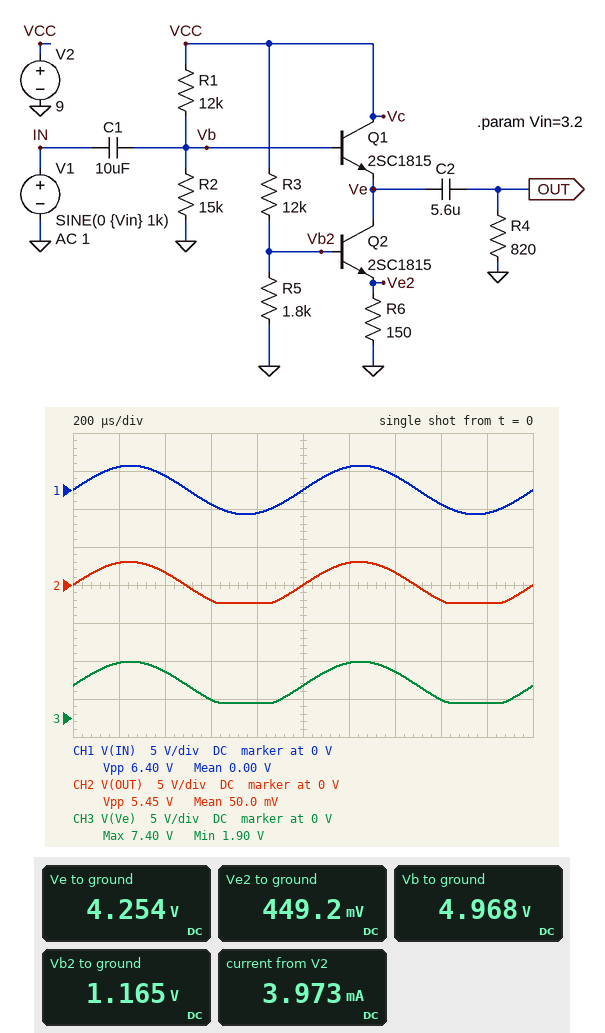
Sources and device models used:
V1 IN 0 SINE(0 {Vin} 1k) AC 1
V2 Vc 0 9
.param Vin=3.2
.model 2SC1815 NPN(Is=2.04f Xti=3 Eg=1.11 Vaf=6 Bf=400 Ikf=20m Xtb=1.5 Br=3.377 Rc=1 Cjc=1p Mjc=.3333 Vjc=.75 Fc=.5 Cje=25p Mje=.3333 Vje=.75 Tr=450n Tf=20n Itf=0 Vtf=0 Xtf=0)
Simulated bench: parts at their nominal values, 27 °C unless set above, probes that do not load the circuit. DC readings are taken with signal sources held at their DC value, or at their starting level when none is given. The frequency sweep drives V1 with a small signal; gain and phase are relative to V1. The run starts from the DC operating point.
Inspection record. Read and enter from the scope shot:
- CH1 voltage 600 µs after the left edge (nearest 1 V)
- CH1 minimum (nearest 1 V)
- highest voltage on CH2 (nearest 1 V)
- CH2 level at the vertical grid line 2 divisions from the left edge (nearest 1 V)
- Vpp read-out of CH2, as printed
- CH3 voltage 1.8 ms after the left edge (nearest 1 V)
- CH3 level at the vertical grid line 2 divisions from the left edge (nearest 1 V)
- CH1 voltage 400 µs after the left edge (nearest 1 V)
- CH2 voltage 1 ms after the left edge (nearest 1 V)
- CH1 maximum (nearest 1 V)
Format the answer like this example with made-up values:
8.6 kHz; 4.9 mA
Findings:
-2 V; -3 V; 3 V; 2 V; 5.45 V; 2 V; 6 V; 2 V; 0 V; 3 V
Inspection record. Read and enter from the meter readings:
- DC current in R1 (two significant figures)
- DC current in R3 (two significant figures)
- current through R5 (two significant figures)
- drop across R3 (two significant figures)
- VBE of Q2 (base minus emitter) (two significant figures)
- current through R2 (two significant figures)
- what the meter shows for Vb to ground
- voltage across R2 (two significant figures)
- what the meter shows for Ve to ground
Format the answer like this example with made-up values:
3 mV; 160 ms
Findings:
340 µA; 650 µA; 650 µA; 7.8 V; 720 mV; 330 µA; 4.968 V; 5.0 V; 4.254 V
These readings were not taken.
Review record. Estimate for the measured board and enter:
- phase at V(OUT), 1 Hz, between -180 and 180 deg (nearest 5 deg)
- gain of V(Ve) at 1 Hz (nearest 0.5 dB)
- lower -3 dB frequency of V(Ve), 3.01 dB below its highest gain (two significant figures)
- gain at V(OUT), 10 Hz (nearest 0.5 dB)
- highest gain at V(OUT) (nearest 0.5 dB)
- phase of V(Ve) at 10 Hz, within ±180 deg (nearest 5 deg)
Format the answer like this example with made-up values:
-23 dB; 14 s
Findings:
155 deg; -8.5 dB; 2.4 Hz; -11.5 dB; 0 dB; 15 deg
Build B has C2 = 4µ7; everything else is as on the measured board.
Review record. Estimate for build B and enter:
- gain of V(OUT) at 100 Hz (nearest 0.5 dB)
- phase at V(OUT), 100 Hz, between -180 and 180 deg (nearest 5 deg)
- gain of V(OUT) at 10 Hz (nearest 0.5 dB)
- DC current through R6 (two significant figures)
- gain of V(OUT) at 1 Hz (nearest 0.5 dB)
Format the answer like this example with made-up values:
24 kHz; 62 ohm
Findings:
-1.0 dB; 25 deg; -13.0 dB; 3.0 mA; -40.5 dB
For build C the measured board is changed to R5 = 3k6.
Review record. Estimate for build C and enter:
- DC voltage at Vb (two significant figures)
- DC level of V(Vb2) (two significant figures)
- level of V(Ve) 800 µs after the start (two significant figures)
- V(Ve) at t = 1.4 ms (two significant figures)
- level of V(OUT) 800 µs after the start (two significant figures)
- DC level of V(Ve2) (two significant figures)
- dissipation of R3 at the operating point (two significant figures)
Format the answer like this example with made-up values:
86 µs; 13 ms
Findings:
4.9 V; 2.0 V; 1.1 V; 6.0 V; -3.1 V; 1.3 V; 4.1 mW
